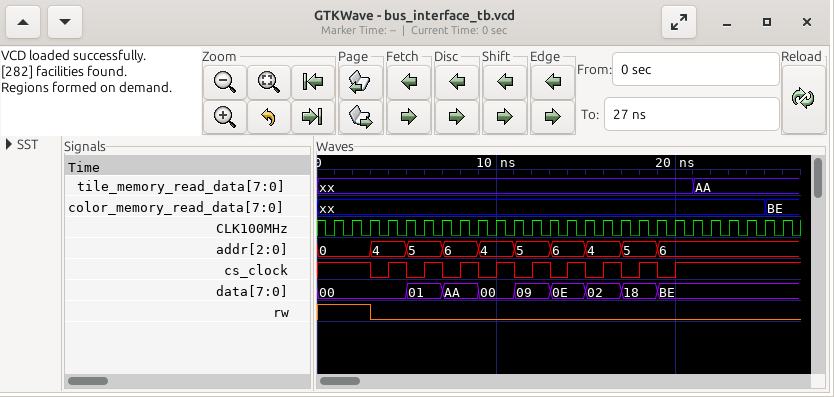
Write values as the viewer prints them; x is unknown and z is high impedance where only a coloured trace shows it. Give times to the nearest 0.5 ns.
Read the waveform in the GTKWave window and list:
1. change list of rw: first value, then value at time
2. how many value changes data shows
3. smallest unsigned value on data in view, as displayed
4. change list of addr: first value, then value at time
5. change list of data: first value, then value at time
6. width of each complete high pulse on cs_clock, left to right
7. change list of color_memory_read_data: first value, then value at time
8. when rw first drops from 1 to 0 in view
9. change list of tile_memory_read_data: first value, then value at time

1, 0 at 3 ns
8
00
0, 4 at 3 ns, 5 at 5 ns, 6 at 7 ns, 4 at 9 ns, 5 at 11 ns, 6 at 13 ns, 4 at 15 ns, 5 at 17 ns, 6 at 19 ns
00, 01 at 5 ns, AA at 7 ns, 00 at 9 ns, 09 at 11 ns, 0E at 13 ns, 02 at 15 ns, 18 at 17 ns, BE at 19 ns
1 ns, 1 ns, 1 ns, 1 ns, 1 ns, 1 ns, 1 ns, 1 ns
xx, BE at 25 ns
3 ns
xx, AA at 21 ns
